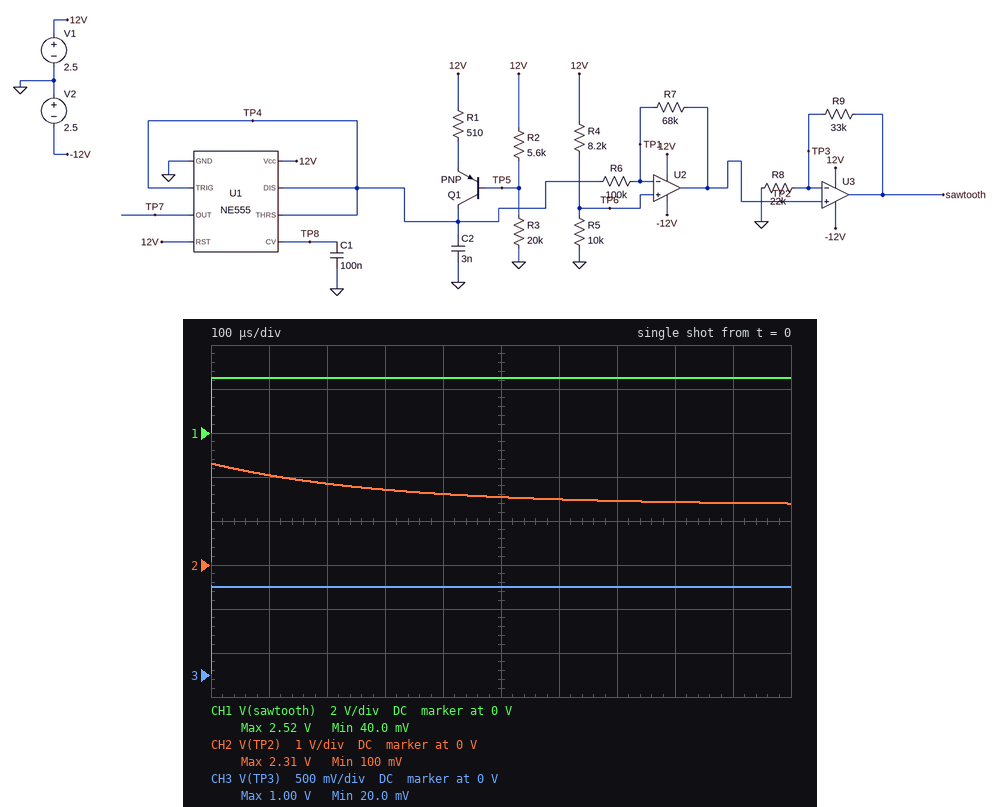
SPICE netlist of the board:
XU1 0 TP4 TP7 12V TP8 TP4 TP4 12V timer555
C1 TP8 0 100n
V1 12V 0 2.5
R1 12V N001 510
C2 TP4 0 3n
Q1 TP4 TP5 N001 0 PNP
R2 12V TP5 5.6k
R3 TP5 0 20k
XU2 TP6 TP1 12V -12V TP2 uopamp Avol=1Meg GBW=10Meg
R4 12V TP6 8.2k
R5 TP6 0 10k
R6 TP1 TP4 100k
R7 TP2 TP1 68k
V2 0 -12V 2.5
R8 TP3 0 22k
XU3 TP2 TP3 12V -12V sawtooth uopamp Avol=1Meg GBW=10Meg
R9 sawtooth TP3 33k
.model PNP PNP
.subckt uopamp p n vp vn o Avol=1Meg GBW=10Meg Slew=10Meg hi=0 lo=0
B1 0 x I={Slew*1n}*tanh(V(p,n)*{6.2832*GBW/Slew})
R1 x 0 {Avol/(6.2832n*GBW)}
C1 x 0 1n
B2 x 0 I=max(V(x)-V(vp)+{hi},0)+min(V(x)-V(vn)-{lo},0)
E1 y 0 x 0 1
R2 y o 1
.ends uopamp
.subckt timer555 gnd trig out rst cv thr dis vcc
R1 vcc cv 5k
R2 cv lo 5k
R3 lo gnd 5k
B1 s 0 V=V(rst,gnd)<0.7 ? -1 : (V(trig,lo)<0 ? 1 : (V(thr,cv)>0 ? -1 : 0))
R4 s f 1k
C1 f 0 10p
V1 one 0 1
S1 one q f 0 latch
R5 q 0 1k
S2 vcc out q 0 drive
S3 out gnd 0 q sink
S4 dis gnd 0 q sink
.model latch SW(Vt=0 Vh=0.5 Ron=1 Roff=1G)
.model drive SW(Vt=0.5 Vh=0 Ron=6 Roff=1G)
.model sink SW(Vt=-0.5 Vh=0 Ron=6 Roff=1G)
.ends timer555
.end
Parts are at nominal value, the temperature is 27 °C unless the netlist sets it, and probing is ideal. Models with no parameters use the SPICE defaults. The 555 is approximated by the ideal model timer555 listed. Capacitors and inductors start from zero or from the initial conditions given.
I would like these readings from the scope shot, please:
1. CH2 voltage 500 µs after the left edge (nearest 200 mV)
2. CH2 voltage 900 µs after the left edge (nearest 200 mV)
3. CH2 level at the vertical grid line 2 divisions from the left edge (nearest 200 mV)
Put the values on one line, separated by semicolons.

1.6 V; 1.4 V; 1.8 V
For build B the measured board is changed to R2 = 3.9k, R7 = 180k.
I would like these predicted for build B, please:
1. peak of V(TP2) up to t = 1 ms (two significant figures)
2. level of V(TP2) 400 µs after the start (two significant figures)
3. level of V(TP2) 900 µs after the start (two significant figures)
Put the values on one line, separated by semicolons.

2.5 V; 2.2 V; 1.5 V
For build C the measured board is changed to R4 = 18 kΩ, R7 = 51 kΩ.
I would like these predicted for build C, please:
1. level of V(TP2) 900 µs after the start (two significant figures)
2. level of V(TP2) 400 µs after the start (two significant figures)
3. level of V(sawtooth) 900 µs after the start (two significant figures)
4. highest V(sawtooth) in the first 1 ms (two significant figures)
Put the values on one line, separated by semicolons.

910 mV; 1.0 V; 2.3 V; 2.5 V
